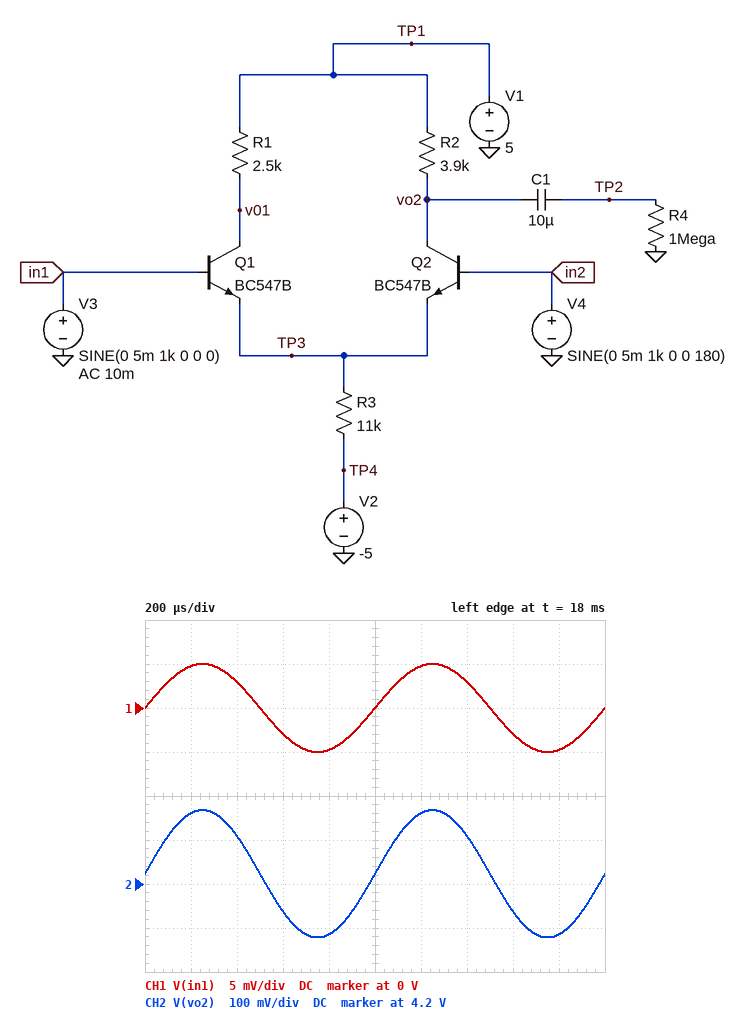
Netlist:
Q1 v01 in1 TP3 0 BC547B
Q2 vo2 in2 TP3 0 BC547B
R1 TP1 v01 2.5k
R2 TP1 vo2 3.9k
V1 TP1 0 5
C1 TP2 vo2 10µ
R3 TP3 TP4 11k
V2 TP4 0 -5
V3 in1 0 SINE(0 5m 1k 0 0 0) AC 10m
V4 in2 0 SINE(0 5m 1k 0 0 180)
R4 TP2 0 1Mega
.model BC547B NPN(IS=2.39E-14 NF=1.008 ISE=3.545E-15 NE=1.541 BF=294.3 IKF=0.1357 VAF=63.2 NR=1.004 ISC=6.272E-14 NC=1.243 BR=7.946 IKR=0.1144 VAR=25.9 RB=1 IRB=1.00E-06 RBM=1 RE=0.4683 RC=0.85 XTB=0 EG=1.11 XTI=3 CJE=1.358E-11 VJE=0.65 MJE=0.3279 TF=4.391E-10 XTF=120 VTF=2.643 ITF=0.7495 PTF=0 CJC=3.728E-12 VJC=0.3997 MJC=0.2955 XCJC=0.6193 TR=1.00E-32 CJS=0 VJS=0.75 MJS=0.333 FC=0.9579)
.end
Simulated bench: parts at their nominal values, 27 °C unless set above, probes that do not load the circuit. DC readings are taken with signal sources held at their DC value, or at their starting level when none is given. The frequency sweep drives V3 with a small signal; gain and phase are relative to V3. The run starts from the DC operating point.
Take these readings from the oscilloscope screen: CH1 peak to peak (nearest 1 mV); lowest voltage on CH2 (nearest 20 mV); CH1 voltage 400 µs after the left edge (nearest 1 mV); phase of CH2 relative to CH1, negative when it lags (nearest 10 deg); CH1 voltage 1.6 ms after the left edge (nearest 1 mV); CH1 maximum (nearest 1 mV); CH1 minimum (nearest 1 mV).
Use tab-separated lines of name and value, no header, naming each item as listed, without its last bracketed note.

CH1 peak to peak	10 mV
lowest voltage on CH2	4.08 V
CH1 voltage 400 µs after the left edge	3 mV
phase of CH2 relative to CH1, negative when it lags	0 deg
CH1 voltage 1.6 ms after the left edge	-3 mV
CH1 maximum	5 mV
CH1 minimum	-5 mV
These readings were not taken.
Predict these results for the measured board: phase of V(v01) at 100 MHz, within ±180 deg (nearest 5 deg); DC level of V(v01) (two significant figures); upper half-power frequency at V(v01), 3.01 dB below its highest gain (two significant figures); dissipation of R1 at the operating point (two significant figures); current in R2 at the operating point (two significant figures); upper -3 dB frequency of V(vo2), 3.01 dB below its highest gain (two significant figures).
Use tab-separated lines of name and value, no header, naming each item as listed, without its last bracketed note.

phase of V(v01) at 100 MHz, within ±180 deg	90 deg
DC level of V(v01)	4.5 V
upper half-power frequency at V(v01), 3.01 dB below its highest gain	36 MHz
dissipation of R1 at the operating point	100 µW
current in R2 at the operating point	200 µA
upper -3 dB frequency of V(vo2), 3.01 dB below its highest gain	23 MHz
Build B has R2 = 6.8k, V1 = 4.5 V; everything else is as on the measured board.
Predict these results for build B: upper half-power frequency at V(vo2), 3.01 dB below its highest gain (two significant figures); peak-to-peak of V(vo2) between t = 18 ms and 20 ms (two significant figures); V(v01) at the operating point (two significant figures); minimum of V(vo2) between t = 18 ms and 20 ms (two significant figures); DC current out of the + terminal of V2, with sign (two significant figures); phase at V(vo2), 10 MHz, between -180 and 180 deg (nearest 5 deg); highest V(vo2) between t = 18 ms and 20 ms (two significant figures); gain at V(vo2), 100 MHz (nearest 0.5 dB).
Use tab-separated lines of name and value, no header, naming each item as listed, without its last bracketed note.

upper half-power frequency at V(vo2), 3.01 dB below its highest gain	12 MHz
peak-to-peak of V(vo2) between t = 18 ms and 20 ms	500 mV
V(v01) at the operating point	4.0 V
minimum of V(vo2) between t = 18 ms and 20 ms	2.9 V
DC current out of the + terminal of V2, with sign	-400 µA
phase at V(vo2), 10 MHz, between -180 and 180 deg	-40 deg
highest V(vo2) between t = 18 ms and 20 ms	3.4 V
gain at V(vo2), 100 MHz	9.5 dB
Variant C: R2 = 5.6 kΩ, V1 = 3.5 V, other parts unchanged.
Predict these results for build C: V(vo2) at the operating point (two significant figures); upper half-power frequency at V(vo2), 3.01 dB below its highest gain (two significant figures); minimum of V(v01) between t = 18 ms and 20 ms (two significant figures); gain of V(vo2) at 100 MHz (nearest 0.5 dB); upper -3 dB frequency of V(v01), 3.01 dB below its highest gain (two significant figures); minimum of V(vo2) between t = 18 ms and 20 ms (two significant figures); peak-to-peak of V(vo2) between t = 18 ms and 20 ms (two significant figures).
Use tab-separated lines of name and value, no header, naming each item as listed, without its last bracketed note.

V(vo2) at the operating point	2.4 V
upper half-power frequency at V(vo2), 3.01 dB below its highest gain	14 MHz
minimum of V(v01) between t = 18 ms and 20 ms	2.9 V
gain of V(vo2) at 100 MHz	9.0 dB
upper -3 dB frequency of V(v01), 3.01 dB below its highest gain	33 MHz
minimum of V(vo2) between t = 18 ms and 20 ms	2.2 V
peak-to-peak of V(vo2) between t = 18 ms and 20 ms	410 mV
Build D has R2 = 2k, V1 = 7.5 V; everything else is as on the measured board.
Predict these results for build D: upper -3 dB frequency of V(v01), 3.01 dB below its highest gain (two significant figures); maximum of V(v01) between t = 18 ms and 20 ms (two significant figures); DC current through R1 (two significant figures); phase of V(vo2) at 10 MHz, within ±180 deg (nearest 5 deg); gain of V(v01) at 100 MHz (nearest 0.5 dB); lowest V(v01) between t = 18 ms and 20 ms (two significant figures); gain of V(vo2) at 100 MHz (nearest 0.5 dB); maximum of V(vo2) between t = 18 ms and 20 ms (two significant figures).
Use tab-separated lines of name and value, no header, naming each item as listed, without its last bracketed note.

upper -3 dB frequency of V(v01), 3.01 dB below its highest gain	41 MHz
maximum of V(v01) between t = 18 ms and 20 ms	7.1 V
DC current through R1	200 µA
phase of V(vo2) at 10 MHz, within ±180 deg	-10 deg
gain of V(v01) at 100 MHz	11.5 dB
lowest V(v01) between t = 18 ms and 20 ms	6.9 V
gain of V(vo2) at 100 MHz	10.5 dB
maximum of V(vo2) between t = 18 ms and 20 ms	7.2 V
